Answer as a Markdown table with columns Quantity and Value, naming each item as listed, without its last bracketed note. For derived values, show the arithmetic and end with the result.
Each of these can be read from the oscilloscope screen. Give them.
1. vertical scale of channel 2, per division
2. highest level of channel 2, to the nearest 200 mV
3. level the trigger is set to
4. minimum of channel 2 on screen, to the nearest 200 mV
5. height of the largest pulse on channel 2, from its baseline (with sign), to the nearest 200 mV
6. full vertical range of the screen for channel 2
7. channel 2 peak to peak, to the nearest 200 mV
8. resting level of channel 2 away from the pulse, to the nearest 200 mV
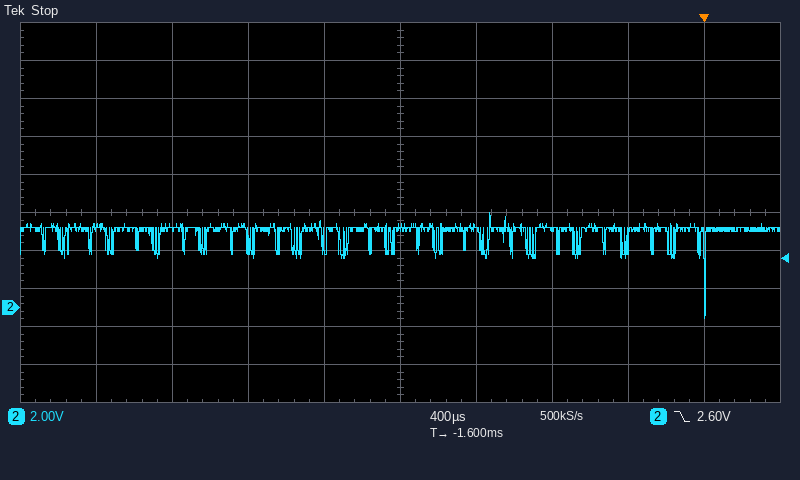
| Quantity | Value |
|---|---|
| vertical scale of channel 2, per division | 2 V |
| highest level of channel 2, to the nearest 200 mV | 5.0 V |
| level the trigger is set to | 2.60 V |
| minimum of channel 2 on screen, to the nearest 200 mV | -600 mV |
| height of the largest pulse on channel 2, from its baseline (with sign), to the nearest 200 mV | -600 mV − (4.2 V) = -4.8 V |
| full vertical range of the screen for channel 2 | 20 V |
| channel 2 peak to peak, to the nearest 200 mV | 5.0 V − (-600 mV) = 5.6 V |
| resting level of channel 2 away from the pulse, to the nearest 200 mV | 4.2 V |
